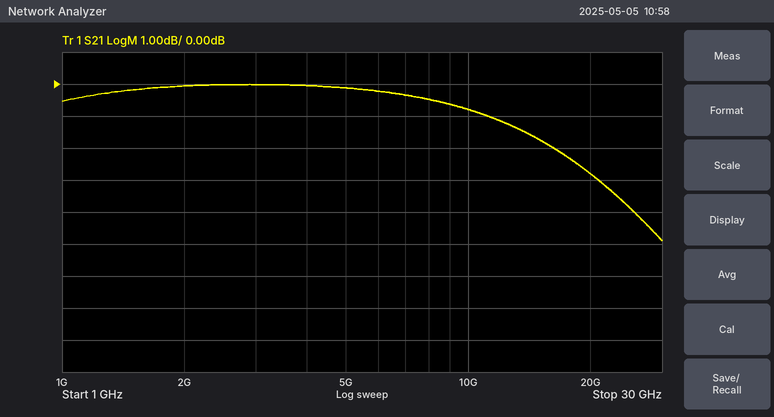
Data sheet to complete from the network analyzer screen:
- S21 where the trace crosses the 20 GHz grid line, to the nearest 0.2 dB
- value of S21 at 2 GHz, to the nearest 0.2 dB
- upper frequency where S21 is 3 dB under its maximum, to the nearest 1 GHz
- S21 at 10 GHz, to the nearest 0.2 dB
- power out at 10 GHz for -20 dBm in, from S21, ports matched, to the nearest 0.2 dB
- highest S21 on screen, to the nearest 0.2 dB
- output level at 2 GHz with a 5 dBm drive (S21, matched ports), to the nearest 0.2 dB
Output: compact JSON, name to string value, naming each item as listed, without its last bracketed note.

{"S21 where the trace crosses the 20 GHz grid line, to the nearest 0.2 dB": "-2.8 dB", "value of S21 at 2 GHz, to the nearest 0.2 dB": "0.0 dB", "upper frequency where S21 is 3 dB under its maximum, to the nearest 1 GHz": "21 GHz", "S21 at 10 GHz, to the nearest 0.2 dB": "-0.8 dB", "power out at 10 GHz for -20 dBm in, from S21, ports matched, to the nearest 0.2 dB": "-20.8 dBm", "highest S21 on screen, to the nearest 0.2 dB": "0.0 dB", "output level at 2 GHz with a 5 dBm drive (S21, matched ports), to the nearest 0.2 dB": "5.0 dBm"}
